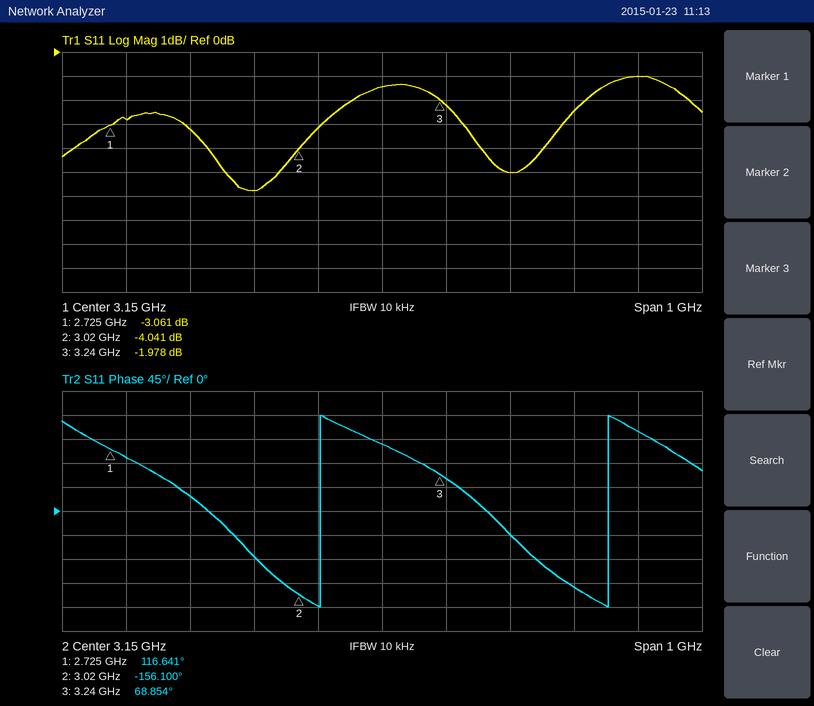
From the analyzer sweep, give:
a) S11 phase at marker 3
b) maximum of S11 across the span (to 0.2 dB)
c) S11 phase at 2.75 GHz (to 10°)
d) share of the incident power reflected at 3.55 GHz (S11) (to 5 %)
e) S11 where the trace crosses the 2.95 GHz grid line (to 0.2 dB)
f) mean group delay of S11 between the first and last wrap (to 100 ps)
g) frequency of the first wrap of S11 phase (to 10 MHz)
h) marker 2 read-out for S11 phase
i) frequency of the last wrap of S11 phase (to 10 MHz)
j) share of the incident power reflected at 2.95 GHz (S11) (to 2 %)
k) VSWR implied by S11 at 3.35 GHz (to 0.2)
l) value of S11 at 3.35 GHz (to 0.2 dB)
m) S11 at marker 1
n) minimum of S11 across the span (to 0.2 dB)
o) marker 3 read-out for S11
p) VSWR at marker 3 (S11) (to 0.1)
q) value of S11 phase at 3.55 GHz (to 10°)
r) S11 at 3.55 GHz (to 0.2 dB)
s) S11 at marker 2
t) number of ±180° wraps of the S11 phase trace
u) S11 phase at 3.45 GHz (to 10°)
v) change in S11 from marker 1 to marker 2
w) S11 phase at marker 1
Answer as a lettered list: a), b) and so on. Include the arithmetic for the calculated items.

a) 68.854°
b) -1.0 dB
c) 100°
d) 10^(-1/10) ≈ 79.4 %, so 80 % to the nearest 5 %
e) -5.8 dB
f) 1 cycle / (3.50 GHz − 3.05 GHz) ≈ 2.2 ns
g) 3.05 GHz
h) -156.100°
i) 3.50 GHz
j) 10^(-5.8/10) ≈ 26 %
k) |Γ| = 10^(-5/20) = 0.5623; VSWR = (1 + 0.5623)/(1 − 0.5623) ≈ 3.6
l) -5.0 dB
m) -3.061 dB
n) -5.8 dB
o) -1.978 dB
p) (1 + 0.7963)/(1 − 0.7963) ≈ 8.8
q) 150°
r) -1.0 dB
s) -4.041 dB
t) 2
u) -140°
v) -4.041 − (-3.061) = -0.980 dB
w) 116.641°
